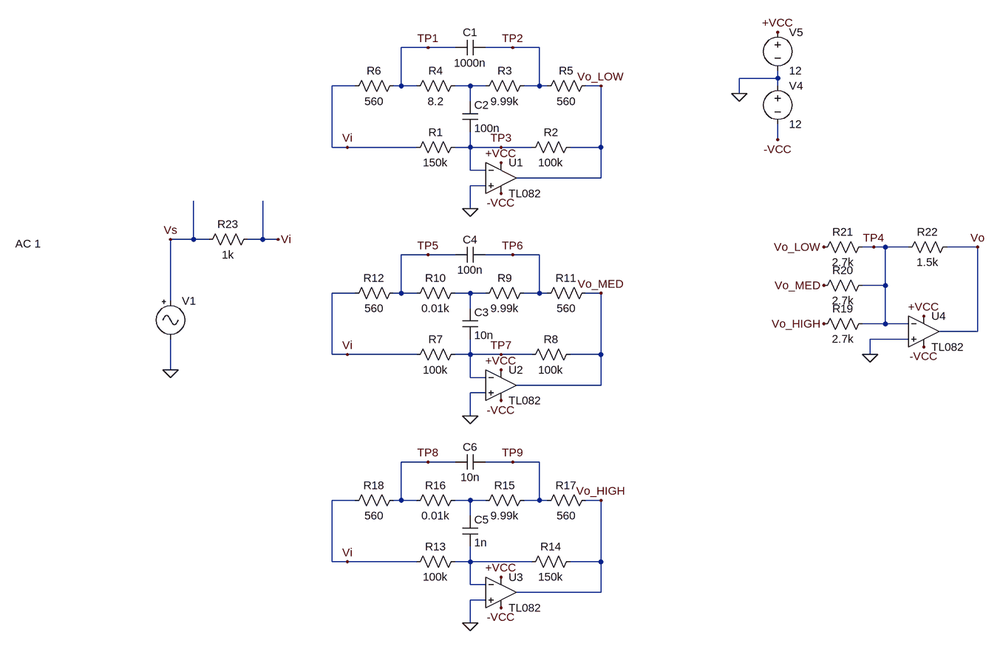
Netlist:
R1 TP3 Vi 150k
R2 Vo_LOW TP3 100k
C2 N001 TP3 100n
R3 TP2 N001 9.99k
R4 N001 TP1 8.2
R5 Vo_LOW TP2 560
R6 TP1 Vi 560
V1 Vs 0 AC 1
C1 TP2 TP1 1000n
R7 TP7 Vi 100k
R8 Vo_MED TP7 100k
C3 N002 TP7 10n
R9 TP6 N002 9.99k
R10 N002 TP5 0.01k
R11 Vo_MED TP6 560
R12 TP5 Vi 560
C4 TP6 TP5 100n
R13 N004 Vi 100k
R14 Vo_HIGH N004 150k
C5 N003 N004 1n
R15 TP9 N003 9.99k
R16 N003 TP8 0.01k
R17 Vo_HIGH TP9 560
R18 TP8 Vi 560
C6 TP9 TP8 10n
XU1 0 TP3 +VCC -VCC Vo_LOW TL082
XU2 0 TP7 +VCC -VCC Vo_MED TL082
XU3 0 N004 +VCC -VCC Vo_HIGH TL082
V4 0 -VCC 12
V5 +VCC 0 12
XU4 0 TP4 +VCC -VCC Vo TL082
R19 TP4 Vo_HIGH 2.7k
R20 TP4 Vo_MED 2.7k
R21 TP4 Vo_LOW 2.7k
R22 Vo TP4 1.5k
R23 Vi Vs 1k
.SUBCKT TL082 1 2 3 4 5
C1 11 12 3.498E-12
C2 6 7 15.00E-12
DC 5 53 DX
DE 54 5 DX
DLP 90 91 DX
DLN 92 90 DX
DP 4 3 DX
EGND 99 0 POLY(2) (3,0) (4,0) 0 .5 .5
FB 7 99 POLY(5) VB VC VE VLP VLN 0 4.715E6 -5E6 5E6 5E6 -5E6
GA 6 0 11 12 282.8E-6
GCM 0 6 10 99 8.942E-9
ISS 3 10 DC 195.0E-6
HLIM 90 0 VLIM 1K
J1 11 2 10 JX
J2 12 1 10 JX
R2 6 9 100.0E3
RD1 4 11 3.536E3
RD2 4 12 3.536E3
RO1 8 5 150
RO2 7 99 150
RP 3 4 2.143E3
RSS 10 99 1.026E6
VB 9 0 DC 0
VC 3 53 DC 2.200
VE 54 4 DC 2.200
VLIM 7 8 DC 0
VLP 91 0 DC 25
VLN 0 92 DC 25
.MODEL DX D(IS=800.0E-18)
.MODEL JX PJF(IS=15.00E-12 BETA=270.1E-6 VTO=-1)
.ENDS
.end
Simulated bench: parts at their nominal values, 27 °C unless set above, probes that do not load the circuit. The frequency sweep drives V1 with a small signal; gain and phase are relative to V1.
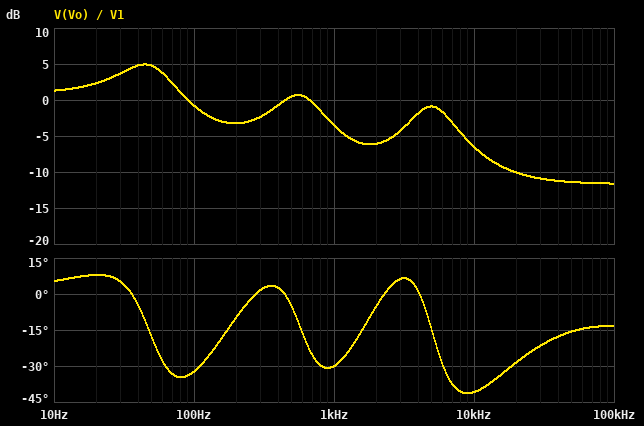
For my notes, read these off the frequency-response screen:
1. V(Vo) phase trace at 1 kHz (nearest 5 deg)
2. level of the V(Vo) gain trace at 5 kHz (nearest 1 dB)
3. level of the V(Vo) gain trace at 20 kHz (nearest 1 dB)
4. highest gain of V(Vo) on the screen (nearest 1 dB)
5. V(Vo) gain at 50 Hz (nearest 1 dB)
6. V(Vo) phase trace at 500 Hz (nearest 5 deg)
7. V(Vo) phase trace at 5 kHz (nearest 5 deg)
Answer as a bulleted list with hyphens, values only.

- -30 deg
- -1 dB
- -10 dB
- 5 dB
- 5 dB
- -5 deg
- -15 deg
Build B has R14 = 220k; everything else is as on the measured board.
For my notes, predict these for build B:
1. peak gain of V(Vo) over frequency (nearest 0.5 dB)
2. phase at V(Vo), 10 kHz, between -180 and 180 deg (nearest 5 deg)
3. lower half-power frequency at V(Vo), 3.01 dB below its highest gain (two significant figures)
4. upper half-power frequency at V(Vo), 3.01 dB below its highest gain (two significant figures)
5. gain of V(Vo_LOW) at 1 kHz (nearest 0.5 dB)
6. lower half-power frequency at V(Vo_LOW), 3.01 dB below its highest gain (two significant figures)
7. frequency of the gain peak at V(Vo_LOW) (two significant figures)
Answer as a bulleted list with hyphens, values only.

- 5.5 dB
- -45 deg
- 9.1 Hz
- 72 Hz
- -15.0 dB
- 31 Hz
- 50 Hz
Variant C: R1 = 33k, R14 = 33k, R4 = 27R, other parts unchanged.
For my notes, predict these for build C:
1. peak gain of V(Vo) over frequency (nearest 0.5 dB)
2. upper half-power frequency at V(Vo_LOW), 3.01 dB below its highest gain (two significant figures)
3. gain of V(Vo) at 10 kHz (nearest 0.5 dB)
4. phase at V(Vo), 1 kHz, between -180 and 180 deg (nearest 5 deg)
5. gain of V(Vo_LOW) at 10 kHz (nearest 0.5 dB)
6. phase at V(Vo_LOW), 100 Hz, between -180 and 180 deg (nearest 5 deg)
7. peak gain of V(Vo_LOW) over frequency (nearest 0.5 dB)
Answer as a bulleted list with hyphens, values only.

- 4.0 dB
- 81 Hz
- -7.0 dB
- -40 deg
- -14.5 dB
- 125 deg
- 7.0 dB
